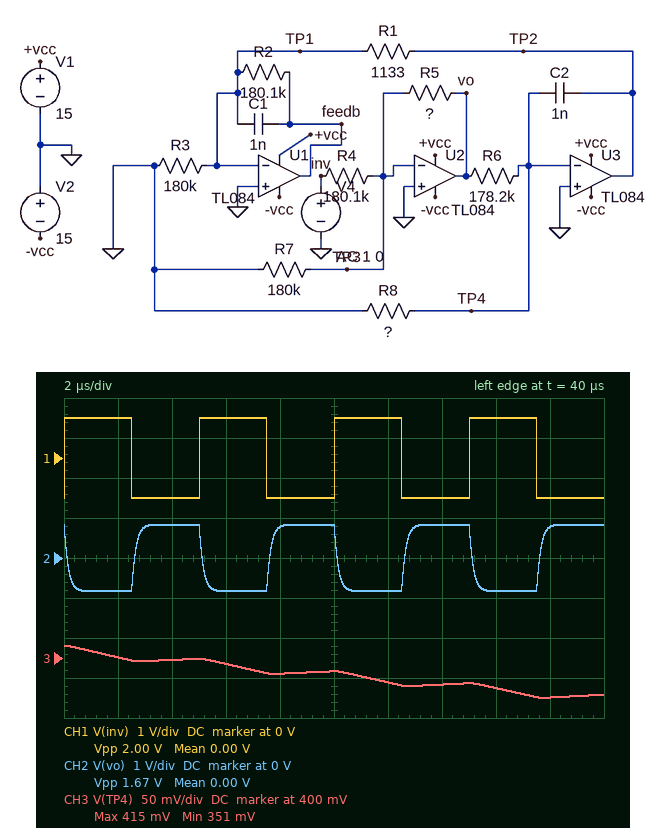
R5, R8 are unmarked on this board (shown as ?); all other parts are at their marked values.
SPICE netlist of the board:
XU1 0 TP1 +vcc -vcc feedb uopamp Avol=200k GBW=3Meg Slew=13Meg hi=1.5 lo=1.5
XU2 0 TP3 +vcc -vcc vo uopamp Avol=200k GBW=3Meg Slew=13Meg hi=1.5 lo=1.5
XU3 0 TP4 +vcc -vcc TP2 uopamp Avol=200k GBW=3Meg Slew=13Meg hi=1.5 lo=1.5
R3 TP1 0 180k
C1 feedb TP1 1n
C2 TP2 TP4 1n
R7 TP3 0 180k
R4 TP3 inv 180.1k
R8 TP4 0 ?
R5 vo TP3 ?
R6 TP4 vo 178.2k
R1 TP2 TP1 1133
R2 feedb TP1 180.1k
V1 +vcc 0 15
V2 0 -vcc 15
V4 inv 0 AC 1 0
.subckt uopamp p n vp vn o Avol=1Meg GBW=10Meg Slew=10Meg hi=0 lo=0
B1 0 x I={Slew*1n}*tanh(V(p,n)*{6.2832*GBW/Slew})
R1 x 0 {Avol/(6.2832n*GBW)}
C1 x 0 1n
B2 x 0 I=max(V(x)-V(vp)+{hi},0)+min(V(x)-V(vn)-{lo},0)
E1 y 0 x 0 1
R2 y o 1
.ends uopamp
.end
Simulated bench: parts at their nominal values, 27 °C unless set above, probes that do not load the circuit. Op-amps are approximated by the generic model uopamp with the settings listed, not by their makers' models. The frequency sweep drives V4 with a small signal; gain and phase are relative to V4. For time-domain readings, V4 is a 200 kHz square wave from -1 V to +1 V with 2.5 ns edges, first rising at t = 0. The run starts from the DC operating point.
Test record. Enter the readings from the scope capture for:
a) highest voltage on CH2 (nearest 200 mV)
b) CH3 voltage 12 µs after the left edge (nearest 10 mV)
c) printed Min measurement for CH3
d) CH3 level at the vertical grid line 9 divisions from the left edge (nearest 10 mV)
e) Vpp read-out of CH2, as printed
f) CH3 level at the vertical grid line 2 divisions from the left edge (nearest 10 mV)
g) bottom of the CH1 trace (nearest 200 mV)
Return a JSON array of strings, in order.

["800 mV", "370 mV", "351 mV", "350 mV", "1.67 V", "400 mV", "-1.0 V"]
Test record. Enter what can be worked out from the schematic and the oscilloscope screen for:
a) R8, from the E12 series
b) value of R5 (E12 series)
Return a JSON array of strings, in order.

["390 kΩ", "150 kΩ"]
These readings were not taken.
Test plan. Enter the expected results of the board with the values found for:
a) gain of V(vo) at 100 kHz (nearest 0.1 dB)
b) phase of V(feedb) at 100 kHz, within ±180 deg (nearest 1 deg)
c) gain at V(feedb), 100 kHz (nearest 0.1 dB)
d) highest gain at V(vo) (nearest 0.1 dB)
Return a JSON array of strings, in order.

["-1.6 dB", "-8 deg", "-40.1 dB", "-1.6 dB"]
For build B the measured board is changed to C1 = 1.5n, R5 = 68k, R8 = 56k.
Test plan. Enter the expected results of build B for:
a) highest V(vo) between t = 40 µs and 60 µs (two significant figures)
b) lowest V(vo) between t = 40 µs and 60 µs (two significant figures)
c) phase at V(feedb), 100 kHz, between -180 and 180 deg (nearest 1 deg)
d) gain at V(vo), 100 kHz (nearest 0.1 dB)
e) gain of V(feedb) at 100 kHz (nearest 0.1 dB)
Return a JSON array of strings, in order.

["380 mV", "-380 mV", "-7 deg", "-8.5 dB", "-50.3 dB"]
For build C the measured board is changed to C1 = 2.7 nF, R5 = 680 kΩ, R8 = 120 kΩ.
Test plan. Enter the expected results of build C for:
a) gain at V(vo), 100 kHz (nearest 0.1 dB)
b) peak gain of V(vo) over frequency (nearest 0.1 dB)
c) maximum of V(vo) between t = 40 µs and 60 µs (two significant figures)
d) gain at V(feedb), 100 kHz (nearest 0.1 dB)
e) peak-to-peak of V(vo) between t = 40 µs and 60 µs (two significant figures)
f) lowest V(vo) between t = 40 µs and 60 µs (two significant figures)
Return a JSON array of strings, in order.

["11.2 dB", "11.5 dB", "3.7 V", "-35.6 dB", "7.5 V", "-3.7 V"]
